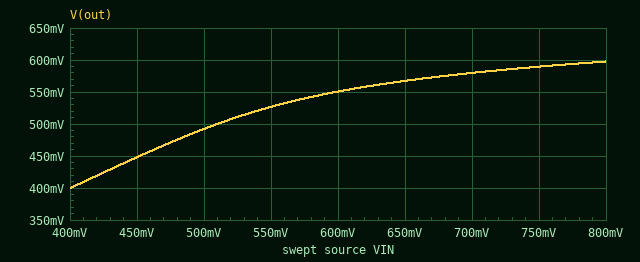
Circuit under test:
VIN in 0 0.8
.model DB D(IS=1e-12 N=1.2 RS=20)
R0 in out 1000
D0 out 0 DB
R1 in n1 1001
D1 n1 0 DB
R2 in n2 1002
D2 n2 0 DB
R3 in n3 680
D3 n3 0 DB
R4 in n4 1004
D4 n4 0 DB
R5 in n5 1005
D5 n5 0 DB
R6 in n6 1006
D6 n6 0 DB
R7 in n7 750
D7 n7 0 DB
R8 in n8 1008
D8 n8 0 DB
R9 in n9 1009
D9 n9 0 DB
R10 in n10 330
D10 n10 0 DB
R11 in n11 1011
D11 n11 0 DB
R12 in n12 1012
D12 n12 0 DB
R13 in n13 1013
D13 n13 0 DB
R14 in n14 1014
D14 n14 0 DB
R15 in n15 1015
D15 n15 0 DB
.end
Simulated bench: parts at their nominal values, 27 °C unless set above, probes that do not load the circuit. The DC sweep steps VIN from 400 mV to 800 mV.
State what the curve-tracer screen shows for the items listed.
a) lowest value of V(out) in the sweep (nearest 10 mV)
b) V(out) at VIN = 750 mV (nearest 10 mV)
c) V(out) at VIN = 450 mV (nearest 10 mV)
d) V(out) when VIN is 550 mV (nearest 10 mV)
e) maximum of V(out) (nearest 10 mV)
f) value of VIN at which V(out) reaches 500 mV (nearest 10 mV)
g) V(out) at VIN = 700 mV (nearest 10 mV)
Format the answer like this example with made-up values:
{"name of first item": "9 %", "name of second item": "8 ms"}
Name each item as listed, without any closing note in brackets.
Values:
{"lowest value of V(out) in the sweep": "400 mV", "V(out) at VIN = 750 mV": "590 mV", "V(out) at VIN = 450 mV": "450 mV", "V(out) when VIN is 550 mV": "530 mV", "maximum of V(out)": "600 mV", "value of VIN at which V(out) reaches 500 mV": "510 mV", "V(out) at VIN = 700 mV": "580 mV"}
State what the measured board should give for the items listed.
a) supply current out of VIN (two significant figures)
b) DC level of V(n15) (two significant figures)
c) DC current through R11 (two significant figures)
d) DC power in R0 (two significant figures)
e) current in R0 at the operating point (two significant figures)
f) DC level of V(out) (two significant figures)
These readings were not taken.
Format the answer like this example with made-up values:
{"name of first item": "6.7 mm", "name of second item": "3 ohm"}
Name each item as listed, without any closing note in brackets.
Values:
{"supply current out of VIN": "3.7 mA", "DC level of V(n15)": "600 mV", "DC current through R11": "200 µA", "DC power in R0": "41 µW", "current in R0 at the operating point": "200 µA", "DC level of V(out)": "600 mV"}
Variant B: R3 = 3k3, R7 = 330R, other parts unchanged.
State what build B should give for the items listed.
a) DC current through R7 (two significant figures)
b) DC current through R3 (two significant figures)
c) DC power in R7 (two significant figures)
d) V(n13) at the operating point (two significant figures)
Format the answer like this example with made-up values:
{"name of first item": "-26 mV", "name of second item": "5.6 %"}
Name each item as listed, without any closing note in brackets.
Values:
{"DC current through R7": "510 µA", "DC current through R3": "72 µA", "DC power in R7": "85 µW", "V(n13) at the operating point": "600 mV"}
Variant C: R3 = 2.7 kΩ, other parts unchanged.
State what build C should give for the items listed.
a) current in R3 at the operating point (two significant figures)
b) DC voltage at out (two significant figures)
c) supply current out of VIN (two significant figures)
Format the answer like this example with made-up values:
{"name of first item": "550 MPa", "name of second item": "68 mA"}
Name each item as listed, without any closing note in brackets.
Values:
{"current in R3 at the operating point": "86 µA", "DC voltage at out": "600 mV", "supply current out of VIN": "3.5 mA"}
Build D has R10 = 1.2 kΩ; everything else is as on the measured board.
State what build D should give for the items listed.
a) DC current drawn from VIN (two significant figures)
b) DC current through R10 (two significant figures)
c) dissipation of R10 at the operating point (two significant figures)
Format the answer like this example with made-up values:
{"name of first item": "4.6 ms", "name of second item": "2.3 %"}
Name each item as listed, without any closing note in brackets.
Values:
{"DC current drawn from VIN": "3.3 mA", "DC current through R10": "170 µA", "dissipation of R10 at the operating point": "36 µW"}
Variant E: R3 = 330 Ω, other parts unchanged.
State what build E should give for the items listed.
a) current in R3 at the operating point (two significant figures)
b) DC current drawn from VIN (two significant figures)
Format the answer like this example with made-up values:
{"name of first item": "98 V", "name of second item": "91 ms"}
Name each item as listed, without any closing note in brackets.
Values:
{"current in R3 at the operating point": "510 µA", "DC current drawn from VIN": "3.9 mA"}
